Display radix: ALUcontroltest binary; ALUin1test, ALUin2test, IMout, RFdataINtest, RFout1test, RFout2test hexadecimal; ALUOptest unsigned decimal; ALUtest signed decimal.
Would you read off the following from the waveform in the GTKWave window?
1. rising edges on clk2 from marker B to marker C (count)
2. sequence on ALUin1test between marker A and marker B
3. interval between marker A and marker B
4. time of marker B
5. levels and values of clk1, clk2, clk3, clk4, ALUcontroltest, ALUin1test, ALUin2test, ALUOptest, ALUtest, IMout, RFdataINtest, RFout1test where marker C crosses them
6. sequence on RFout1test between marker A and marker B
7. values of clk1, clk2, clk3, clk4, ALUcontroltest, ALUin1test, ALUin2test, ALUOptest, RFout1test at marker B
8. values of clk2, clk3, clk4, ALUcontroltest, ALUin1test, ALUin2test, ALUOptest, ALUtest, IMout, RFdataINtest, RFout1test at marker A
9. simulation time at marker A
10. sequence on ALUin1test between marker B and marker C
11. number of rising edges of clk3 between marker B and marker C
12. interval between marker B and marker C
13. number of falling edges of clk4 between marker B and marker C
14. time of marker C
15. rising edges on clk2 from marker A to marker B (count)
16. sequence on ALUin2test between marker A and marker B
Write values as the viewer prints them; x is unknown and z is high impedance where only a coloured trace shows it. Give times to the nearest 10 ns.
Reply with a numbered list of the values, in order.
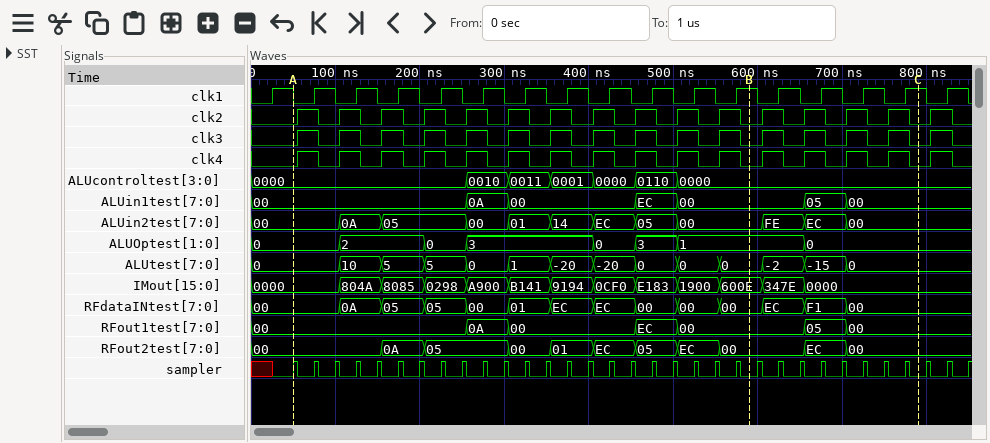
1. 4
2. 00, 0A, 00, EC, 00
3. 540 ns
4. 590 ns
5. clk1=1, clk2=0, clk3=0, clk4=0, ALUcontroltest=0000, ALUin1test=00, ALUin2test=00, ALUOptest=0, ALUtest=0, IMout=0000, RFdataINtest=00, RFout1test=00
6. 00, 0A, 00, EC, 00
7. clk1=1, clk2=0, clk3=0, clk4=0, ALUcontroltest=0000, ALUin1test=00, ALUin2test=00, ALUOptest=1, RFout1test=00
8. clk2=0, clk3=0, clk4=0, ALUcontroltest=0000, ALUin1test=00, ALUin2test=00, ALUOptest=0, ALUtest=0, IMout=0000, RFdataINtest=00, RFout1test=00
9. 50 ns
10. 00, 05, 00
11. 4
12. 200 ns
13. 4
14. 790 ns
15. 11
16. 00, 0A, 05, 00, 01, 14, EC, 05, 00
